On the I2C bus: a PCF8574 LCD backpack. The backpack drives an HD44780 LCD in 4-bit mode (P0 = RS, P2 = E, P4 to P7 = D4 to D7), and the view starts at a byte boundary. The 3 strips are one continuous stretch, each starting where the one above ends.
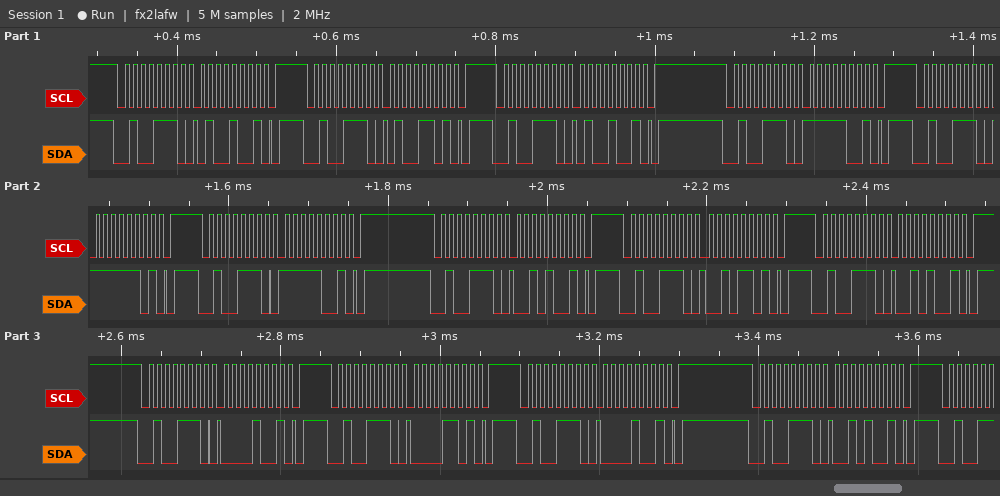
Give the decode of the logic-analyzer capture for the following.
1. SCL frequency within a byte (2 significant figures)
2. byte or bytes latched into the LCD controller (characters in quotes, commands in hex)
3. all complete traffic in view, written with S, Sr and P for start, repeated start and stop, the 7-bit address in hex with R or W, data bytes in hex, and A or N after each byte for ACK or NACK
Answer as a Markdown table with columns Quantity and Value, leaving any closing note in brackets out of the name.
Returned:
| Quantity | Value |
|---|---|
| SCL frequency within a byte | 100 kHz |
| byte or bytes latched into the LCD controller | 'O' ' ' |
| all complete traffic in view, written with S, Sr and P for start, repeated start and stop, the 7-bit address in hex with R or W, data bytes in hex, and A or N after each byte for ACK or NACK | S 27W A 49 A P S 27W A 4D A P S 27W A 49 A P S 27W A F9 A P S 27W A FD A P S 27W A F9 A P S 27W A 29 A P S 27W A 2D A P S 27W A 29 A P S 27W A 09 A P S 27W A 0D A P S 27W A 09 A P S 27W A 29 A P |
